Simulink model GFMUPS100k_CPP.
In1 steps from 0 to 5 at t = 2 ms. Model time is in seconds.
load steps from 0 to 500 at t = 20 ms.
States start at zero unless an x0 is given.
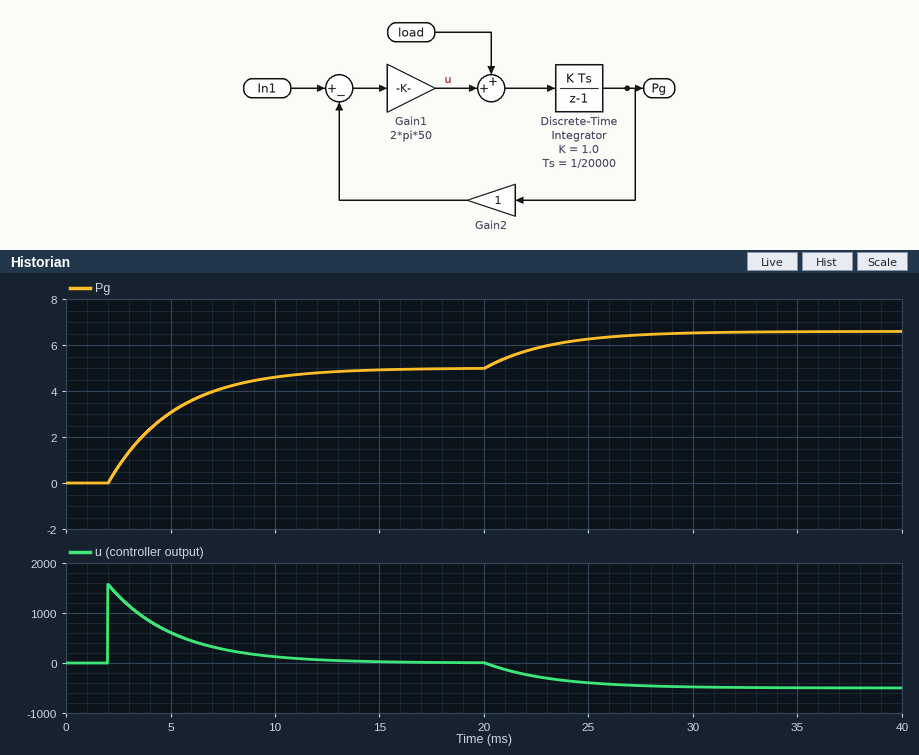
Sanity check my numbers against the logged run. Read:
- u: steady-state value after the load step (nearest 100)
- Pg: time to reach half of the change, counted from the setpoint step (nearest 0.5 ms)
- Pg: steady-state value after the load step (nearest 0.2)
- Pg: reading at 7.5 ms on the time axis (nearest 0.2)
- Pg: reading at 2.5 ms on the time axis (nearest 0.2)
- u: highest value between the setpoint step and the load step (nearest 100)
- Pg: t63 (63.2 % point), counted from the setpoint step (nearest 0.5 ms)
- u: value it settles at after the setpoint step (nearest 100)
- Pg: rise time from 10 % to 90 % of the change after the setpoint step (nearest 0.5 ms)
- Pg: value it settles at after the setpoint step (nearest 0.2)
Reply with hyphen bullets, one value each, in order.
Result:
- -500
- 2.0 ms
- 6.6
- 4.2
- 0.8
- 1600
- 3.0 ms
- 0
- 7.0 ms
- 5.0
